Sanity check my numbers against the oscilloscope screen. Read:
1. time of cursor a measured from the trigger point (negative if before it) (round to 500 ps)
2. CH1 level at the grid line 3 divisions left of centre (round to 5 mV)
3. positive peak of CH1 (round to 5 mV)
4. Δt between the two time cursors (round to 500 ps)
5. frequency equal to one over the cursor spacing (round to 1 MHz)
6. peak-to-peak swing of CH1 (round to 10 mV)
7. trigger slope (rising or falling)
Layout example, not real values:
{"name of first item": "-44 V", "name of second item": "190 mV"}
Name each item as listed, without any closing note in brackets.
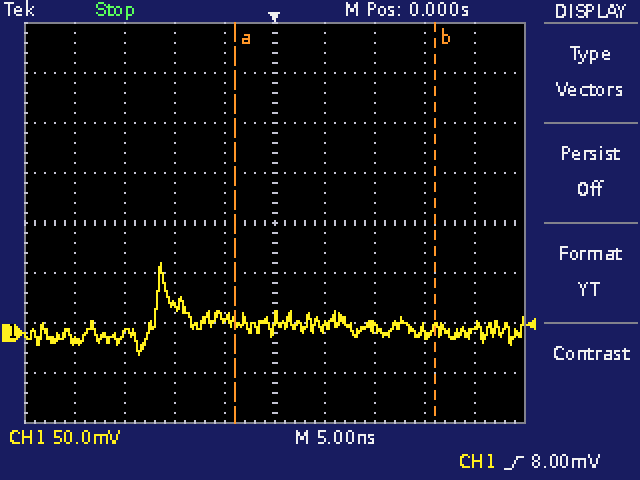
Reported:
{"time of cursor a measured from the trigger point (negative if before it)": "-4.0 ns", "CH1 level at the grid line 3 divisions left of centre": "0 mV", "positive peak of CH1": "70 mV", "Δt between the two time cursors": "20.0 ns", "frequency equal to one over the cursor spacing": "50 MHz", "peak-to-peak swing of CH1": "90 mV", "trigger slope": "rising"}
